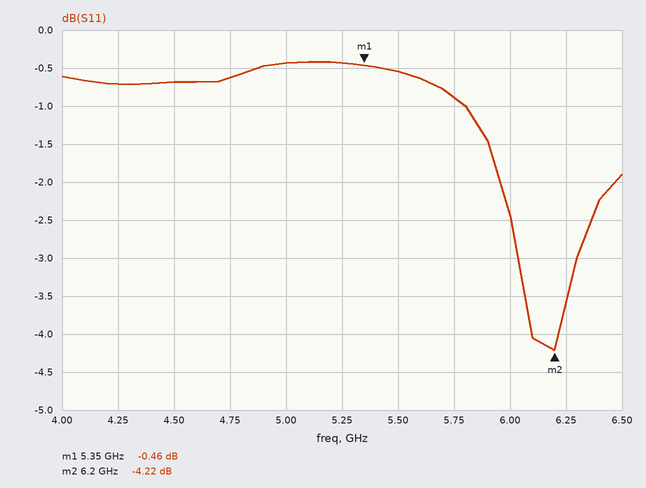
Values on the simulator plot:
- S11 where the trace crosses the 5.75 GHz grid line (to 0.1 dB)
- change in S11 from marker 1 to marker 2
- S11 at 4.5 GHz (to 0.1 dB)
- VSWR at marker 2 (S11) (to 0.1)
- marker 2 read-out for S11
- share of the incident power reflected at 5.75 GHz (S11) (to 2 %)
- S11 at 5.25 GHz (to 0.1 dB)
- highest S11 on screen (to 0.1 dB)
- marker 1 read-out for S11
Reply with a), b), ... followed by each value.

a) -0.9 dB
b) -3.76 dB
c) -0.7 dB
d) 4.2
e) -4.22 dB
f) 82 %
g) -0.4 dB
h) -0.4 dB
i) -0.46 dB
